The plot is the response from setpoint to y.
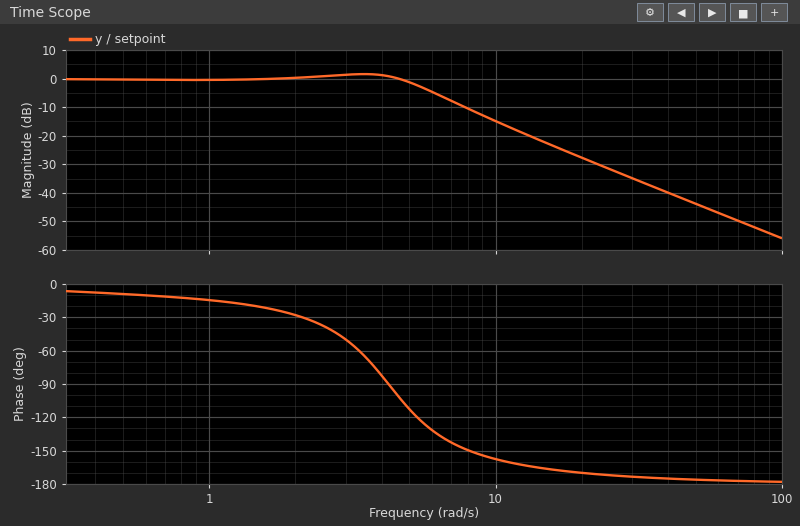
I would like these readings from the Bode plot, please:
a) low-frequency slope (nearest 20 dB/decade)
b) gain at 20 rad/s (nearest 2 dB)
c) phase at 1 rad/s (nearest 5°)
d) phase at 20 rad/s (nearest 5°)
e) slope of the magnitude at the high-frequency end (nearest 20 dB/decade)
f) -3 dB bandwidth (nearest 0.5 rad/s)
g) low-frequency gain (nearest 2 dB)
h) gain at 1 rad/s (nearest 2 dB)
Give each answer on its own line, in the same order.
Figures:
0 dB/decade
-28 dB
-15°
-170°
-40 dB/decade
5.5 rad/s
0 dB
0 dB
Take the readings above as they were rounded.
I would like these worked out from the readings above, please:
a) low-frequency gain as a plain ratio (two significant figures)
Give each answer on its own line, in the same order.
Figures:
1.0
